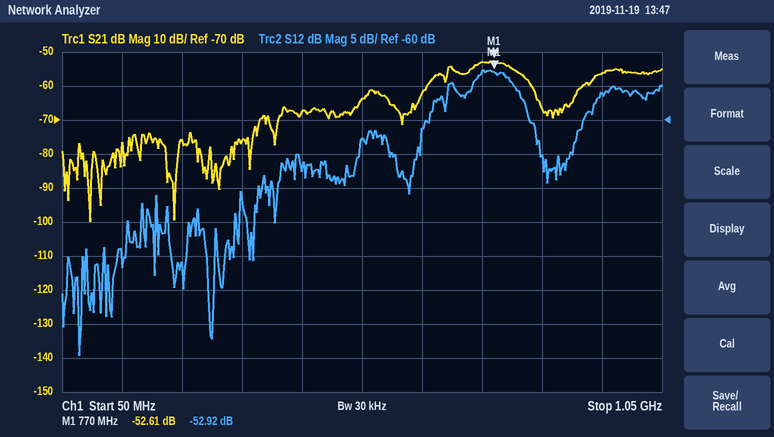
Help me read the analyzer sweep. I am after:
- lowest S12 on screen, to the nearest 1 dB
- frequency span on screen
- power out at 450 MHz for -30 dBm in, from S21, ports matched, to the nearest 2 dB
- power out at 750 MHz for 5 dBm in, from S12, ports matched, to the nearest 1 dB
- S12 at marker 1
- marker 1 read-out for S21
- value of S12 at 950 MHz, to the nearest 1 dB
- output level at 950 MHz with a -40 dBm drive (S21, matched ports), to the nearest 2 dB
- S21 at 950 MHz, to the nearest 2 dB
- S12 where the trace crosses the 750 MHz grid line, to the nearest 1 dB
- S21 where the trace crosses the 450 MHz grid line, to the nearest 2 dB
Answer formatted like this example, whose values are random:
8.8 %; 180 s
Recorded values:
-95 dB; 1 GHz; -98 dBm; -48 dBm; -52.92 dB; -52.61 dB; -56 dB; -96 dBm; -56 dB; -53 dB; -68 dB
